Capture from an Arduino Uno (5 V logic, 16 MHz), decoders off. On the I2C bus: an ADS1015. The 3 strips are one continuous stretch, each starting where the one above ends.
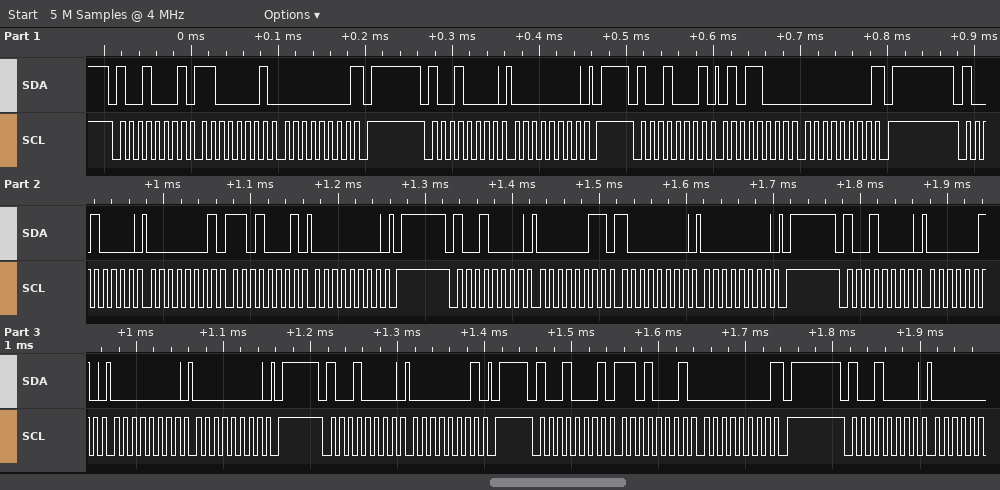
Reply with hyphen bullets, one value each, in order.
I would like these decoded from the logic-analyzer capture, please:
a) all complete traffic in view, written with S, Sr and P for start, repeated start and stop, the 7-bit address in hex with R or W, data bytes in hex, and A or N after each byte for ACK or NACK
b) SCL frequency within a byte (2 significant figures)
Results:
- S 48R A C1 A 00 N P S 48W A 00 A P S 48R A 58 A 00 N P S 48W A 01 A D1 A 00 A P S 48W A 03 A 80 A 00 A P S 48W A 02 A 00 A 00 A P S 48W A 01 A P S 48R A D1 A 00 N P S 48W A
- 100 kHz
